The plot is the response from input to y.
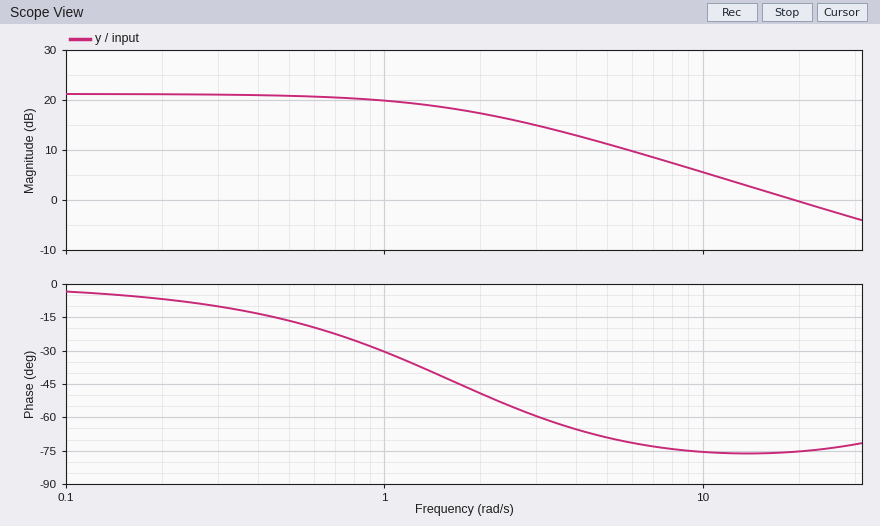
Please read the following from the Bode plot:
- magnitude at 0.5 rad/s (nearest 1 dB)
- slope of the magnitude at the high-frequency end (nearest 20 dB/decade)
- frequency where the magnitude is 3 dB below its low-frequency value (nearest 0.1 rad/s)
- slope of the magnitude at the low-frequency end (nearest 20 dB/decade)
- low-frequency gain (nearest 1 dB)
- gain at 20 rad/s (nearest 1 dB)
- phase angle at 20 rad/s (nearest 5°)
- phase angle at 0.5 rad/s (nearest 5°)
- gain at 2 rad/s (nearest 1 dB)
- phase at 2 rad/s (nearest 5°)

21 dB
-20 dB/decade
1.7 rad/s
0 dB/decade
21 dB
0 dB
-75°
-15°
17 dB
-50°
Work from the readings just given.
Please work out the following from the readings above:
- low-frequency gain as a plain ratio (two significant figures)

11
